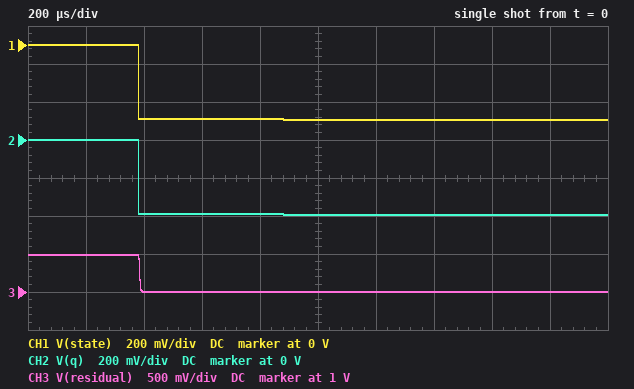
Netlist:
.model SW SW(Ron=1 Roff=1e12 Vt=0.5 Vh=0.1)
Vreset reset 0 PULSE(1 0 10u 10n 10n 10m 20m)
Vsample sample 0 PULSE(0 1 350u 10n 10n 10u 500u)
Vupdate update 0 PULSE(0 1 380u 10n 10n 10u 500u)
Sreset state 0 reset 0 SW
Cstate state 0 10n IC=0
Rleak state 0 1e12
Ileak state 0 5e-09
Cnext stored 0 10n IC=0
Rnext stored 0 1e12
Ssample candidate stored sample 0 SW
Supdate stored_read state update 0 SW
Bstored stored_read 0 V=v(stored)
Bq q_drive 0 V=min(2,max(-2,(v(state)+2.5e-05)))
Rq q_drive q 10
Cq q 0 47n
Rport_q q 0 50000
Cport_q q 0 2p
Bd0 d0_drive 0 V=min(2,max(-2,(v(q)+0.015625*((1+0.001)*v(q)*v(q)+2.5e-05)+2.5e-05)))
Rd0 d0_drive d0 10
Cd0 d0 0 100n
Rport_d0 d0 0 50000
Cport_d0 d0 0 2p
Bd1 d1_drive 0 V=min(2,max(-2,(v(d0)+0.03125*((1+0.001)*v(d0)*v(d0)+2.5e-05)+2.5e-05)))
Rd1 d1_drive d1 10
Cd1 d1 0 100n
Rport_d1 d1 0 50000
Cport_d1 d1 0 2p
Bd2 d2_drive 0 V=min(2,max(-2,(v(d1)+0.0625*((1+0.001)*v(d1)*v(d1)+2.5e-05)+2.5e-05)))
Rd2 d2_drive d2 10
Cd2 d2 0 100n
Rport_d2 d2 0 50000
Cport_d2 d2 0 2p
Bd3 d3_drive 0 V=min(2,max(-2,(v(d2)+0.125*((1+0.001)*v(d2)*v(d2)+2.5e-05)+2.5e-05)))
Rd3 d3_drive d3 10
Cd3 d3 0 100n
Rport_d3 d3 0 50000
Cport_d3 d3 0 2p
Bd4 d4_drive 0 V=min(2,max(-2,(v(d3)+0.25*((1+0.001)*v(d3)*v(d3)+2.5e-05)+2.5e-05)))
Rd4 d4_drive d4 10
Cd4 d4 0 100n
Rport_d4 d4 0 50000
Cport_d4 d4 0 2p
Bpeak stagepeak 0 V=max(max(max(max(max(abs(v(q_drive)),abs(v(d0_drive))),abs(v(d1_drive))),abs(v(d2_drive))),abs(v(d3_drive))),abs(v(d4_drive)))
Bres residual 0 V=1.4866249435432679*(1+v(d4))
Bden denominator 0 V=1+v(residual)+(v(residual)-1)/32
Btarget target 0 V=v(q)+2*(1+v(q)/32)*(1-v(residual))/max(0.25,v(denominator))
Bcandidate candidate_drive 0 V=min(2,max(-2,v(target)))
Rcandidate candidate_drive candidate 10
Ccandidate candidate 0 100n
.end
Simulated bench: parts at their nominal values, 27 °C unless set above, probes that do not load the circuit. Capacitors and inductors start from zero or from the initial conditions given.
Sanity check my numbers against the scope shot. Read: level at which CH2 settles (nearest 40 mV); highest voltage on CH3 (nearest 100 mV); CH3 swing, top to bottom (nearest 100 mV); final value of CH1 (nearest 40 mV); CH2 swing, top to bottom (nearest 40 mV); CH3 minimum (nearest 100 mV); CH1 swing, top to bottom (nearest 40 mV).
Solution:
-400 mV
1.5 V
500 mV
-400 mV
400 mV
1.0 V
400 mV
